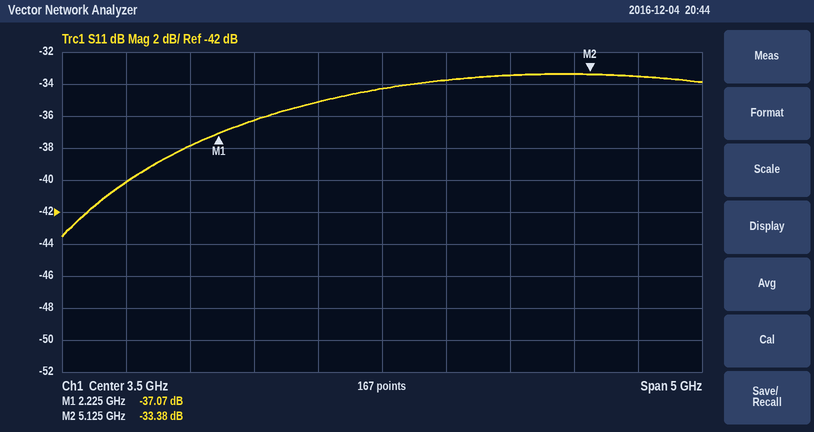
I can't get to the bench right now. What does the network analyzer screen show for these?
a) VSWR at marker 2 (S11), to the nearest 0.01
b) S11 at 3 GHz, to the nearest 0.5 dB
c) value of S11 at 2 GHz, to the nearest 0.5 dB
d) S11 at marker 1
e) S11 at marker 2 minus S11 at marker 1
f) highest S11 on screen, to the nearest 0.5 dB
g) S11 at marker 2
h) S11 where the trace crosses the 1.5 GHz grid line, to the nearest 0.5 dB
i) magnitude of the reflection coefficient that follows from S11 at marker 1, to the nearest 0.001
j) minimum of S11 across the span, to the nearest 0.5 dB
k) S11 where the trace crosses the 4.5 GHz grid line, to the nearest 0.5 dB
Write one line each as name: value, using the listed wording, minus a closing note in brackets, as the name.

VSWR at marker 2 (S11), to the nearest 0.01: 1.04
S11 at 3 GHz, to the nearest 0.5 dB: -35.0 dB
value of S11 at 2 GHz, to the nearest 0.5 dB: -38.0 dB
S11 at marker 1: -37.07 dB
S11 at marker 2 minus S11 at marker 1: 3.69 dB
highest S11 on screen, to the nearest 0.5 dB: -33.5 dB
S11 at marker 2: -33.38 dB
S11 where the trace crosses the 1.5 GHz grid line, to the nearest 0.5 dB: -40.0 dB
magnitude of the reflection coefficient that follows from S11 at marker 1, to the nearest 0.001: 0.014
minimum of S11 across the span, to the nearest 0.5 dB: -43.5 dB
S11 where the trace crosses the 4.5 GHz grid line, to the nearest 0.5 dB: -33.5 dB
